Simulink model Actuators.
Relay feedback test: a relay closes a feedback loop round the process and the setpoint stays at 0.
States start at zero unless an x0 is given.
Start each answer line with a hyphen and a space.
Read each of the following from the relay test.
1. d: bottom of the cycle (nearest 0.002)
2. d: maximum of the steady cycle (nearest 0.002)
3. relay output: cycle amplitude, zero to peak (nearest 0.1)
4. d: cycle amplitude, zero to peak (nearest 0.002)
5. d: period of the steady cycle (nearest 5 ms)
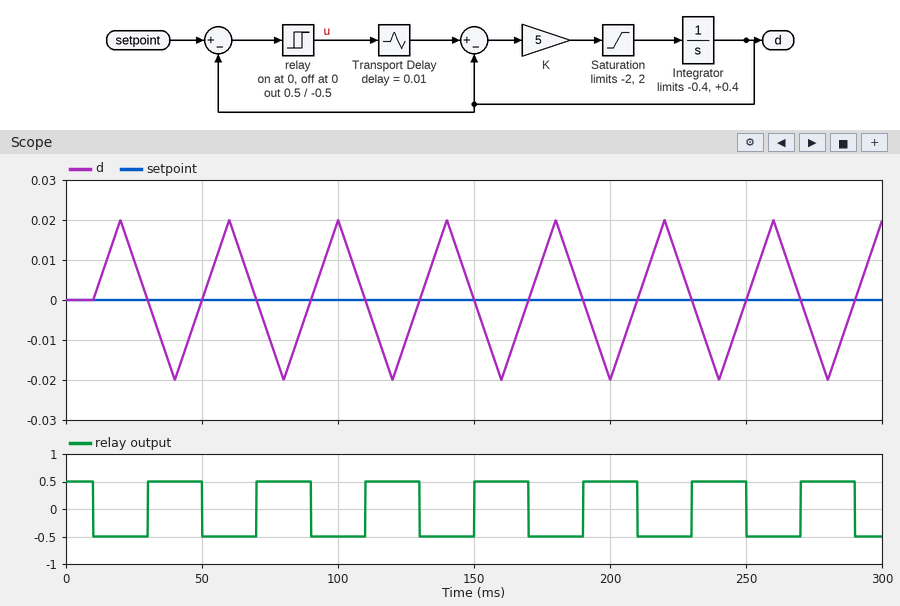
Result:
- -0.020
- 0.020
- 0.5
- 0.020
- 40 ms
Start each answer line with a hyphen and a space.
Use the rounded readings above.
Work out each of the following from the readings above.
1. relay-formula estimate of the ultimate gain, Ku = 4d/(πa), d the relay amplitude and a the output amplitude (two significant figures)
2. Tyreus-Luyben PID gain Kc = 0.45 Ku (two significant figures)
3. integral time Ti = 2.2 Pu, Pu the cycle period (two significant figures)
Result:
- 32
- 14
- 88 ms
